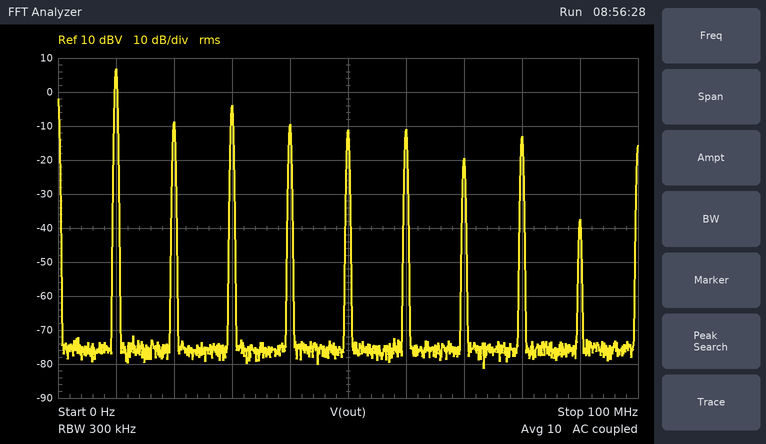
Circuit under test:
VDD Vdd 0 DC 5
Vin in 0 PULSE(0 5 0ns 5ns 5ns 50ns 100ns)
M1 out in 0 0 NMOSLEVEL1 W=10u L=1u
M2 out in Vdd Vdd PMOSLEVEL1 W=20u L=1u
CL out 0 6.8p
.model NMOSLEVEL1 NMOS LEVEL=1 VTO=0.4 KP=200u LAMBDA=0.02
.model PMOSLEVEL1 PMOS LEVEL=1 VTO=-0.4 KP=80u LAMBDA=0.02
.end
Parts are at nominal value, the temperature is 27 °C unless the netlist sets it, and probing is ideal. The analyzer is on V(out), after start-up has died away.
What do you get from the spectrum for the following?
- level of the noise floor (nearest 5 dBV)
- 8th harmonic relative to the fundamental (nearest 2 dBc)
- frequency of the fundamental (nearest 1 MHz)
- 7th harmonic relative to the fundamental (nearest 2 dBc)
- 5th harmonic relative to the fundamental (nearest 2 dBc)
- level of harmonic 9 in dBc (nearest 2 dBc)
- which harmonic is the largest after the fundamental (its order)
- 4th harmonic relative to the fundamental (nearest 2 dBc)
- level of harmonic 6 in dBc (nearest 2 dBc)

-75 dBV
-20 dBc
10 MHz
-26 dBc
-18 dBc
-44 dBc
3
-16 dBc
-18 dBc
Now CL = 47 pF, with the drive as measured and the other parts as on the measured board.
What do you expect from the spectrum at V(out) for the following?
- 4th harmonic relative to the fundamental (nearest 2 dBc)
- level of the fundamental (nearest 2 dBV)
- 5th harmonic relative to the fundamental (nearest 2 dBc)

-22 dBc
6 dBV
-26 dBc
